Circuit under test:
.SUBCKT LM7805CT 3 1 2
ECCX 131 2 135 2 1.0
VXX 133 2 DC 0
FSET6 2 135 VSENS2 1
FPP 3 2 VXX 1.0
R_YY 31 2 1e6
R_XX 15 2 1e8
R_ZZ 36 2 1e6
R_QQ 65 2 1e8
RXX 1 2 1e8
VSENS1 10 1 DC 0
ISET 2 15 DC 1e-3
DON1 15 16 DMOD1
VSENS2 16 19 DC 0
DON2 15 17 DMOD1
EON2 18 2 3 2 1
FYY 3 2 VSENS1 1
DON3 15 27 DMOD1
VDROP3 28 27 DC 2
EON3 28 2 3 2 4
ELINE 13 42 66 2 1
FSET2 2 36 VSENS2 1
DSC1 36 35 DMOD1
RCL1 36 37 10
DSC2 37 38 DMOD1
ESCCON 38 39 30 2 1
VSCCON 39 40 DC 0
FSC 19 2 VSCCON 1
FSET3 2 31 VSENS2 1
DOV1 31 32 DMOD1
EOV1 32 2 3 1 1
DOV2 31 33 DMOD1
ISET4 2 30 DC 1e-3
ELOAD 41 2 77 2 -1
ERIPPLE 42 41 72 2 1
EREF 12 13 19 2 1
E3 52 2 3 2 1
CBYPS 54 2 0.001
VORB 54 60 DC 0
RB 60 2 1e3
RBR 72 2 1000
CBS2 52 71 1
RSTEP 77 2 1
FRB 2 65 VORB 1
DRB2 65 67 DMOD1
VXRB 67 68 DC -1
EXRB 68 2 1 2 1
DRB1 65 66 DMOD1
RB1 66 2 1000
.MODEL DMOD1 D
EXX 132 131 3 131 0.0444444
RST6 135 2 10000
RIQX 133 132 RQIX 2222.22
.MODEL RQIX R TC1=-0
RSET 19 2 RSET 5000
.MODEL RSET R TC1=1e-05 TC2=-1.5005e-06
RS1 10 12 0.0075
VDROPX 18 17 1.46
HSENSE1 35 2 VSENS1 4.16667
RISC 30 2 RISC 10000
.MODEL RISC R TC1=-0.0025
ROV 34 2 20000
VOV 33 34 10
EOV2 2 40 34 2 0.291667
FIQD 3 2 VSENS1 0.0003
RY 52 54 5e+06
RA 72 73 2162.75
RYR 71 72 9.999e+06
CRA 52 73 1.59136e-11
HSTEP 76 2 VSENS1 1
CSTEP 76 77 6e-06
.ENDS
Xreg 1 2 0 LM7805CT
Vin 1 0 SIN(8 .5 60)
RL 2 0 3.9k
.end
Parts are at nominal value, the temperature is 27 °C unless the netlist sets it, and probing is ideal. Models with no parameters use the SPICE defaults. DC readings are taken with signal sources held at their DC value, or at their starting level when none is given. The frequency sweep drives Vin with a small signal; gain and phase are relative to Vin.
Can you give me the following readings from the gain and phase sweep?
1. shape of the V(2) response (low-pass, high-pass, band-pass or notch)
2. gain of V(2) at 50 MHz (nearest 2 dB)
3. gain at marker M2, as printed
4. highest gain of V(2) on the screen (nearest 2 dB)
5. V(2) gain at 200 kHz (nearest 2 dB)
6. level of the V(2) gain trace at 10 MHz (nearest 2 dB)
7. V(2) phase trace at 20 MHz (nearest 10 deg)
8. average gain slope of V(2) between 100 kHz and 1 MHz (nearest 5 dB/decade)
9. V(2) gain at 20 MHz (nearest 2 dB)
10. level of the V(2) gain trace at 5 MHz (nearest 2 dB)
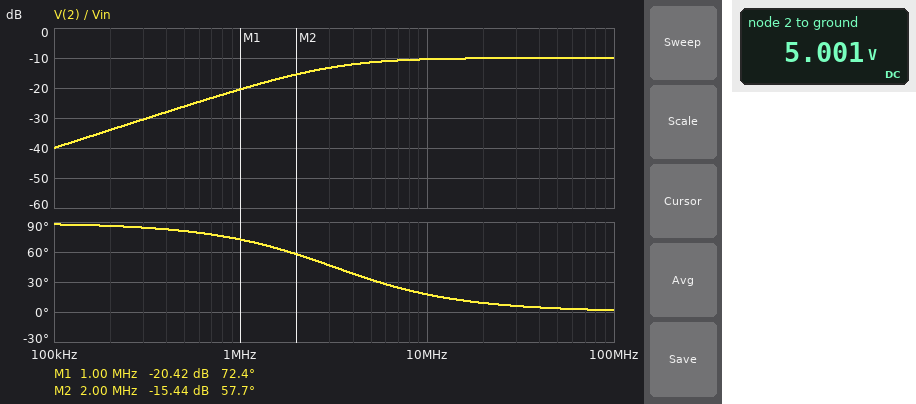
high-pass
-10 dB
-15.44 dB
-10 dB
-34 dB
-10 dB
10 deg
20 dB/decade
-10 dB
-12 dB
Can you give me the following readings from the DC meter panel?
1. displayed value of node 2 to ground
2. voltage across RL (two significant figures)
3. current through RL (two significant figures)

5.001 V
5.0 V
1.3 mA
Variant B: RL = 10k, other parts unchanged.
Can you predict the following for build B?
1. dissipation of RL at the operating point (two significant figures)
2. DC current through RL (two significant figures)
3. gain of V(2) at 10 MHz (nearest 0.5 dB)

2.5 mW
500 µA
-10.5 dB
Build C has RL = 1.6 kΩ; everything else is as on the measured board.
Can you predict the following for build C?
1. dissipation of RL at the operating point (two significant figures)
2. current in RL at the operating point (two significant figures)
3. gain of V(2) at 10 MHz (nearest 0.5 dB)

16 mW
3.1 mA
-10.5 dB
